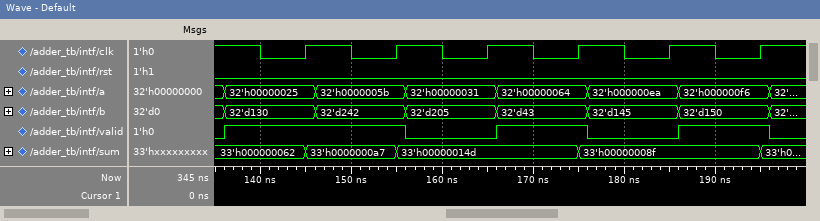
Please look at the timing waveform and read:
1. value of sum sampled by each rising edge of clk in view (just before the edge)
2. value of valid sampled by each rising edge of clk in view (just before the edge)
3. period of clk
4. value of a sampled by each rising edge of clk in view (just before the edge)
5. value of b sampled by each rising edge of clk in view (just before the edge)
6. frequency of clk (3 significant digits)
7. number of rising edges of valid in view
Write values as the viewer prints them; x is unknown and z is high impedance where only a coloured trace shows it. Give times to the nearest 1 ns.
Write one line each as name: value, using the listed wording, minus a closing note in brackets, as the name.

value of sum sampled by each rising edge of clk in view: 33'h000000062, 33'h0000000a7, 33'h00000014d, 33'h00000014d, 33'h00000008f, 33'h00000008f
value of valid sampled by each rising edge of clk in view: 1 1 0 1 0 1
period of clk: 10 ns
value of a sampled by each rising edge of clk in view: 32'h00000025, 32'h0000005b, 32'h00000031, 32'h00000064, 32'h000000ea, 32'h000000f6
value of b sampled by each rising edge of clk in view: 32'd130, 32'd242, 32'd205, 32'd43, 32'd145, 32'd150
frequency of clk: 100 MHz
number of rising edges of valid in view: 3
